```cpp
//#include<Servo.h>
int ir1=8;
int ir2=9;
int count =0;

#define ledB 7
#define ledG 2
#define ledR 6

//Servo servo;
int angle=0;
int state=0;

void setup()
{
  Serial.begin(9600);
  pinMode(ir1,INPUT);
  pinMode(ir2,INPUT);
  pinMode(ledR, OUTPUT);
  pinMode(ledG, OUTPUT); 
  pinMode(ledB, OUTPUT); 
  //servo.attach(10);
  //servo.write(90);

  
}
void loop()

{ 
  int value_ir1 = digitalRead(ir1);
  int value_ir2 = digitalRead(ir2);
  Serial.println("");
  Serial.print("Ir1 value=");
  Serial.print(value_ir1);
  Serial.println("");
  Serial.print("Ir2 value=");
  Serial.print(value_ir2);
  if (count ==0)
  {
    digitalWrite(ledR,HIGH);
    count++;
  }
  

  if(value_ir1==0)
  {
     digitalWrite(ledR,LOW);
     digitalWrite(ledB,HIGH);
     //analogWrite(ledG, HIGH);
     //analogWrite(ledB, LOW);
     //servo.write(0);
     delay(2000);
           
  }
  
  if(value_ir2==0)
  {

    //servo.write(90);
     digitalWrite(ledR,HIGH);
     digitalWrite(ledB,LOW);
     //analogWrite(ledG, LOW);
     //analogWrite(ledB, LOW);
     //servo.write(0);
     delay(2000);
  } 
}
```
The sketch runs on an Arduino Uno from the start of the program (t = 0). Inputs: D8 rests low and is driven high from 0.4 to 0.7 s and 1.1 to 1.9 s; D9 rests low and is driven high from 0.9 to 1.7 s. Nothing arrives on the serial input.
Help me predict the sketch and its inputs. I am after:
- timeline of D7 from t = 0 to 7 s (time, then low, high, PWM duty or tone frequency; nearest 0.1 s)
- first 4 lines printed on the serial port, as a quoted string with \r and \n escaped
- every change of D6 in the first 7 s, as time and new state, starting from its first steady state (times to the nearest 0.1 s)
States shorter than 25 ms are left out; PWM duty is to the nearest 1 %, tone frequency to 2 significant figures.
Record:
0 s high; 2 s low; 4 s high; 6 s low
"\r\nIr1 value=0\r\nIr2 value=0\r\nIr1 value=0\r\n"
0 s low; 2 s high; 4 s low; 6 s high
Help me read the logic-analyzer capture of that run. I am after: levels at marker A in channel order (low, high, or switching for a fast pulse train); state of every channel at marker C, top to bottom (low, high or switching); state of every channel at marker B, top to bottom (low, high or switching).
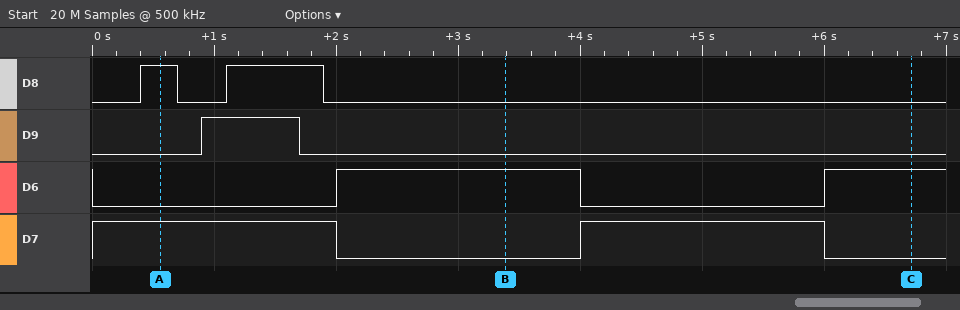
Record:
D8 high, D9 low, D6 low, D7 high
D8 low, D9 low, D6 high, D7 low
D8 low, D9 low, D6 high, D7 low
